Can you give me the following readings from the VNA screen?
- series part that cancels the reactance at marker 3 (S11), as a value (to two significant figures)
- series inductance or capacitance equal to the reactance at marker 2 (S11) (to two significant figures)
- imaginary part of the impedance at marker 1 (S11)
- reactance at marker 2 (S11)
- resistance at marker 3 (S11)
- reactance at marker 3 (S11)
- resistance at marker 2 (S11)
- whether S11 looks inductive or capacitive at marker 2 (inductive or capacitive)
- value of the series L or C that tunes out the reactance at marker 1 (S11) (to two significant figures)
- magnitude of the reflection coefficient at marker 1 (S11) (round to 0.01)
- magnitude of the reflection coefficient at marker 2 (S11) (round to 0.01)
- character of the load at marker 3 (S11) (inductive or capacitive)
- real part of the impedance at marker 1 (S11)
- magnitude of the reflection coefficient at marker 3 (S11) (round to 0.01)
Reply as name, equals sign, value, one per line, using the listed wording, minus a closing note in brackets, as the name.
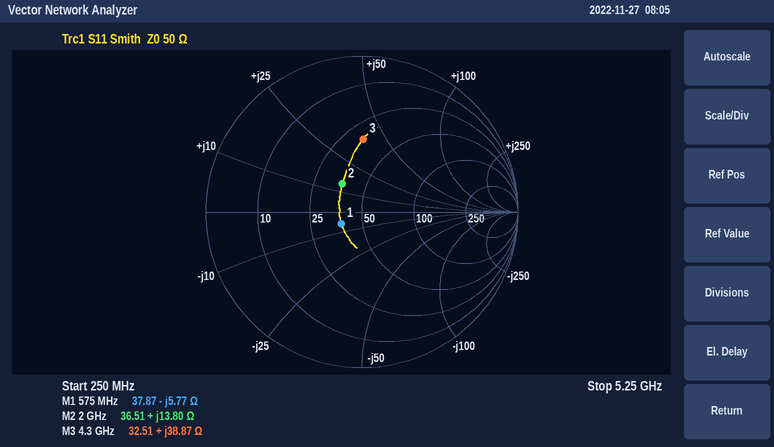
series part that cancels the reactance at marker 3 (S11), as a value = 950 fF
series inductance or capacitance equal to the reactance at marker 2 (S11) = 1.1 nH
imaginary part of the impedance at marker 1 = -5.77 Ω
reactance at marker 2 = +13.80 Ω
resistance at marker 3 = 32.51 Ω
reactance at marker 3 = +38.87 Ω
resistance at marker 2 = 36.51 Ω
whether S11 looks inductive or capacitive at marker 2 = inductive
value of the series L or C that tunes out the reactance at marker 1 (S11) = 1.6 nH
magnitude of the reflection coefficient at marker 1 (S11) = 0.15
magnitude of the reflection coefficient at marker 2 (S11) = 0.22
character of the load at marker 3 (S11) = inductive
real part of the impedance at marker 1 = 37.87 Ω
magnitude of the reflection coefficient at marker 3 (S11) = 0.47
